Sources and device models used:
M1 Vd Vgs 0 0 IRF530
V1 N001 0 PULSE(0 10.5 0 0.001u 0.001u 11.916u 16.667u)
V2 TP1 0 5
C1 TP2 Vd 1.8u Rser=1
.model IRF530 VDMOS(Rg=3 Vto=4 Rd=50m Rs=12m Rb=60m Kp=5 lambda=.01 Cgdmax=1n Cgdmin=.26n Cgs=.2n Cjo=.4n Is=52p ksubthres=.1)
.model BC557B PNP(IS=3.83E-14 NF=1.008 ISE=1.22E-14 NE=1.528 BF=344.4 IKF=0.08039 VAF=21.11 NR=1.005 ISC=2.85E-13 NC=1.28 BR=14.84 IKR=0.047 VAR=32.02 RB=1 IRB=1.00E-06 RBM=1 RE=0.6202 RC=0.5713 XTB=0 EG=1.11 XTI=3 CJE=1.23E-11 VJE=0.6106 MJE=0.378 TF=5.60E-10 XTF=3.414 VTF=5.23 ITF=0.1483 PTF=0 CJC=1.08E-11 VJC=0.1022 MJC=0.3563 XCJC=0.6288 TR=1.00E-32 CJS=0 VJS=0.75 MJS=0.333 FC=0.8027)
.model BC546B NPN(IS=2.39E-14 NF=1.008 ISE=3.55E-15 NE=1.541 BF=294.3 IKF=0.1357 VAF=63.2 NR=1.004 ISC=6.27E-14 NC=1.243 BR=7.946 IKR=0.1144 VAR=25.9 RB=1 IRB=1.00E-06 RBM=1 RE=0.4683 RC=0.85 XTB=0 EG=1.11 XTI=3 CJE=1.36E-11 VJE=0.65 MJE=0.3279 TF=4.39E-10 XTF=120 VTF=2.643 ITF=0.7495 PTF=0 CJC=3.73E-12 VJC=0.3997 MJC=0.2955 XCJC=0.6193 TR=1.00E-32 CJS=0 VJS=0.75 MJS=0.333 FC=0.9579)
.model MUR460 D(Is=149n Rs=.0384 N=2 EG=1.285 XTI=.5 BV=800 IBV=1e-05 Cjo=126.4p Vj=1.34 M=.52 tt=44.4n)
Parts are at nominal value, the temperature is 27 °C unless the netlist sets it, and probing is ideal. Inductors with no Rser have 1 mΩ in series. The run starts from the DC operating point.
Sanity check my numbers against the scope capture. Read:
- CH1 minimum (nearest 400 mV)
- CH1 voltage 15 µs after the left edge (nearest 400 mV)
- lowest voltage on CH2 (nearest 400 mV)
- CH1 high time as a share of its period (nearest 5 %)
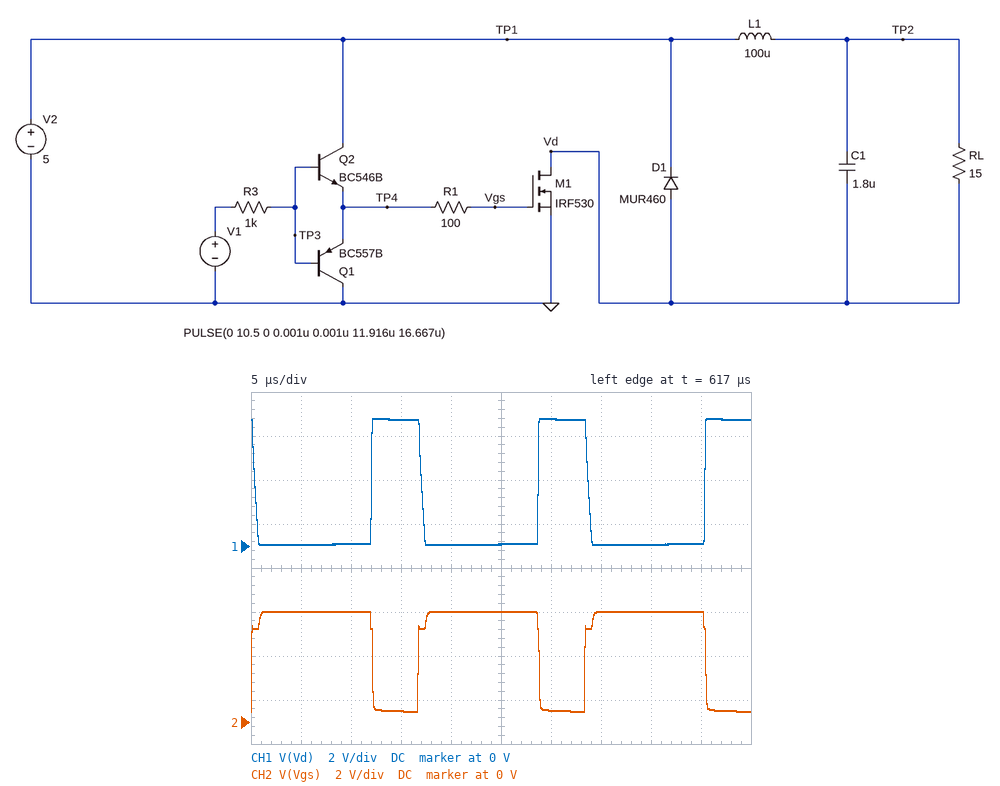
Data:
0 V
5.6 V
400 mV
30 %
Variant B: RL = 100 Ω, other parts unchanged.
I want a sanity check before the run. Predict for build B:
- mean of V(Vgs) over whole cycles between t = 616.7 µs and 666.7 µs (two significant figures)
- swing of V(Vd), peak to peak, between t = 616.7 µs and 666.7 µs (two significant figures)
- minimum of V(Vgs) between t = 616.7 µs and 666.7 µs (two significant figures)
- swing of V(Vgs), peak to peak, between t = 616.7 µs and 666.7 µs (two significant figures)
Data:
3.6 V
6.2 V
-1.3 V
6.3 V
